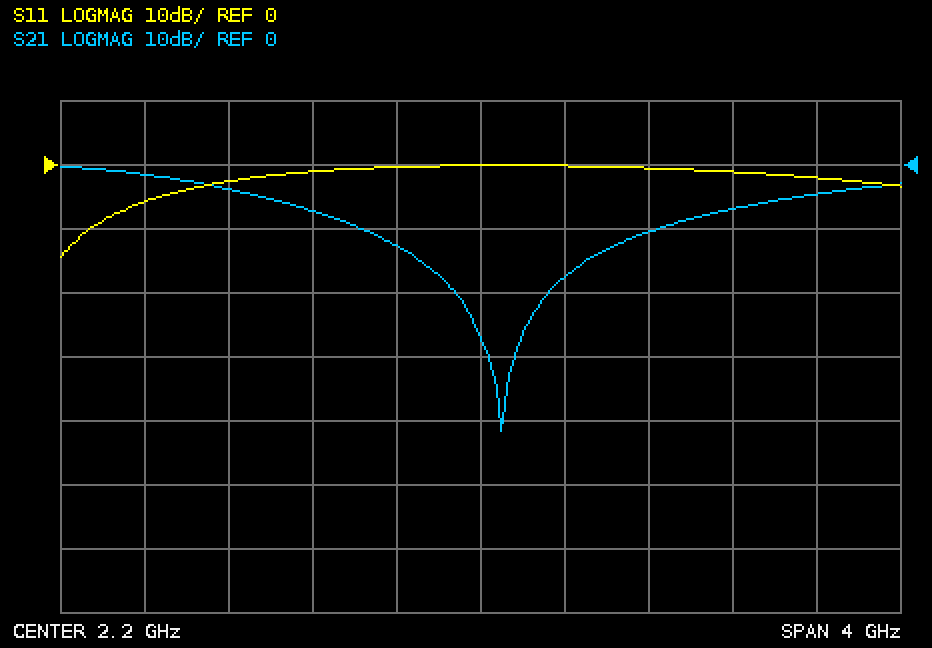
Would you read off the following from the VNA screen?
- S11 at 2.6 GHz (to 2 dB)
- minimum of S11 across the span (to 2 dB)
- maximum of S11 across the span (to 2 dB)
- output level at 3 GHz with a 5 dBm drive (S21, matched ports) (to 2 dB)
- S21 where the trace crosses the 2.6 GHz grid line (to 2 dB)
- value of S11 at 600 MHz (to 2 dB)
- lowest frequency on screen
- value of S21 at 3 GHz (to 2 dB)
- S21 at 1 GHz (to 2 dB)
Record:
0 dB
-14 dB
0 dB
-6 dBm
-18 dB
-6 dB
200 MHz
-10 dB
-4 dB
